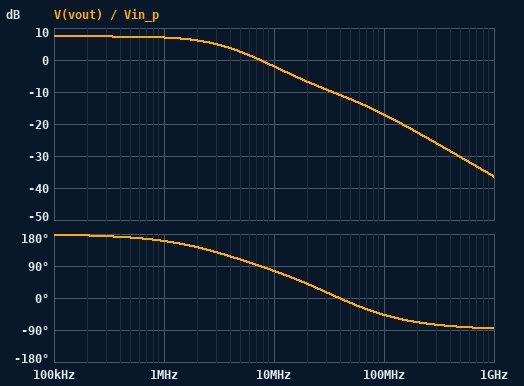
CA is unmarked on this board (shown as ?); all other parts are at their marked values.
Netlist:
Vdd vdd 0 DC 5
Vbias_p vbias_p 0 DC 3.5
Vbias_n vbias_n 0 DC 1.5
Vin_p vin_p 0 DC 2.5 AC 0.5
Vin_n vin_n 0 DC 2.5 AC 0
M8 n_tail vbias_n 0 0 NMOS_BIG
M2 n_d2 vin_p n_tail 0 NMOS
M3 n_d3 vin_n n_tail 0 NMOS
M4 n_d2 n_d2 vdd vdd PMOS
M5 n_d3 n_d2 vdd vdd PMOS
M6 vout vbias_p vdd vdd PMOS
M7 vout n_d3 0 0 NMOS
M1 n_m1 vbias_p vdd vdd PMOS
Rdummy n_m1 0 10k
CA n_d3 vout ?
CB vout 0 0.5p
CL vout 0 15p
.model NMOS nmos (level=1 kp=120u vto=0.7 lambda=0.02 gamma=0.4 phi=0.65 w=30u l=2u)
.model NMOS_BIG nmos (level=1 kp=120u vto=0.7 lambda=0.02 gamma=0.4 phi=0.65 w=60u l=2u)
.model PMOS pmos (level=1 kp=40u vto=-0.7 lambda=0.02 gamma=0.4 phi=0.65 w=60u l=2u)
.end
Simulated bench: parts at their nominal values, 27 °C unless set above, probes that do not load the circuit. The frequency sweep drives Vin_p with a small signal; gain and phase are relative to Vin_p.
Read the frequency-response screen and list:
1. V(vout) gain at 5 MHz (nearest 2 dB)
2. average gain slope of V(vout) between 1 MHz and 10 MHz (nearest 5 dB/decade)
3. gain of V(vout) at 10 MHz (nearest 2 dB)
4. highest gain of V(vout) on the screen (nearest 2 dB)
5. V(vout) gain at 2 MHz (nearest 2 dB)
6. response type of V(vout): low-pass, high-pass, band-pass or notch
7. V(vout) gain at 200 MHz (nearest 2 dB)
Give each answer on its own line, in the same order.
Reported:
2 dB
-10 dB/decade
-2 dB
8 dB
6 dB
low-pass
-22 dB
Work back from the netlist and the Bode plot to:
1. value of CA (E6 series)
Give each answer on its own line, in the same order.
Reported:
1 pF
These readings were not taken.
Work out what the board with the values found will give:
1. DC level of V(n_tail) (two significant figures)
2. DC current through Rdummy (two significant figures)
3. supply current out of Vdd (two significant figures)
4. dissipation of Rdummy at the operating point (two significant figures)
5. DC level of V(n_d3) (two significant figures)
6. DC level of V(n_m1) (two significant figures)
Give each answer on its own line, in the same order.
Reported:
850 mV
390 µA
2.0 mA
1.5 mW
3.3 V
3.9 V
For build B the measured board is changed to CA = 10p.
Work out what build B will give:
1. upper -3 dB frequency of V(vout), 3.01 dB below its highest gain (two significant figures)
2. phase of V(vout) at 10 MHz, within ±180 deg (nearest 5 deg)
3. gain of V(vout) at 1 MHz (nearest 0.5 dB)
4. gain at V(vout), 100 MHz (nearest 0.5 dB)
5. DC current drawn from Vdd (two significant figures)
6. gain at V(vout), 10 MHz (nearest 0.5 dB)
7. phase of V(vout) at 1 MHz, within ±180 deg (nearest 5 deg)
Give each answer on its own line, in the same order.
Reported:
350 kHz
5 deg
-2.0 dB
-17.5 dB
2.0 mA
-10.0 dB
85 deg
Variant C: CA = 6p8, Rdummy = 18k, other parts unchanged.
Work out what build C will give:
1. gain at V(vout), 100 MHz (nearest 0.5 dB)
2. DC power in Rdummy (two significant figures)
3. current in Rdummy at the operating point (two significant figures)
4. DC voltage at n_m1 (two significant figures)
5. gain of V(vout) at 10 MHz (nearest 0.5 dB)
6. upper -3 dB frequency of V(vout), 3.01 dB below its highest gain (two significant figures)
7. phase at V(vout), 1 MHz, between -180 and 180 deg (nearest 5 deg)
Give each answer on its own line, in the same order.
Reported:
-17.5 dB
1.2 mW
260 µA
4.7 V
-10.0 dB
510 kHz
100 deg
